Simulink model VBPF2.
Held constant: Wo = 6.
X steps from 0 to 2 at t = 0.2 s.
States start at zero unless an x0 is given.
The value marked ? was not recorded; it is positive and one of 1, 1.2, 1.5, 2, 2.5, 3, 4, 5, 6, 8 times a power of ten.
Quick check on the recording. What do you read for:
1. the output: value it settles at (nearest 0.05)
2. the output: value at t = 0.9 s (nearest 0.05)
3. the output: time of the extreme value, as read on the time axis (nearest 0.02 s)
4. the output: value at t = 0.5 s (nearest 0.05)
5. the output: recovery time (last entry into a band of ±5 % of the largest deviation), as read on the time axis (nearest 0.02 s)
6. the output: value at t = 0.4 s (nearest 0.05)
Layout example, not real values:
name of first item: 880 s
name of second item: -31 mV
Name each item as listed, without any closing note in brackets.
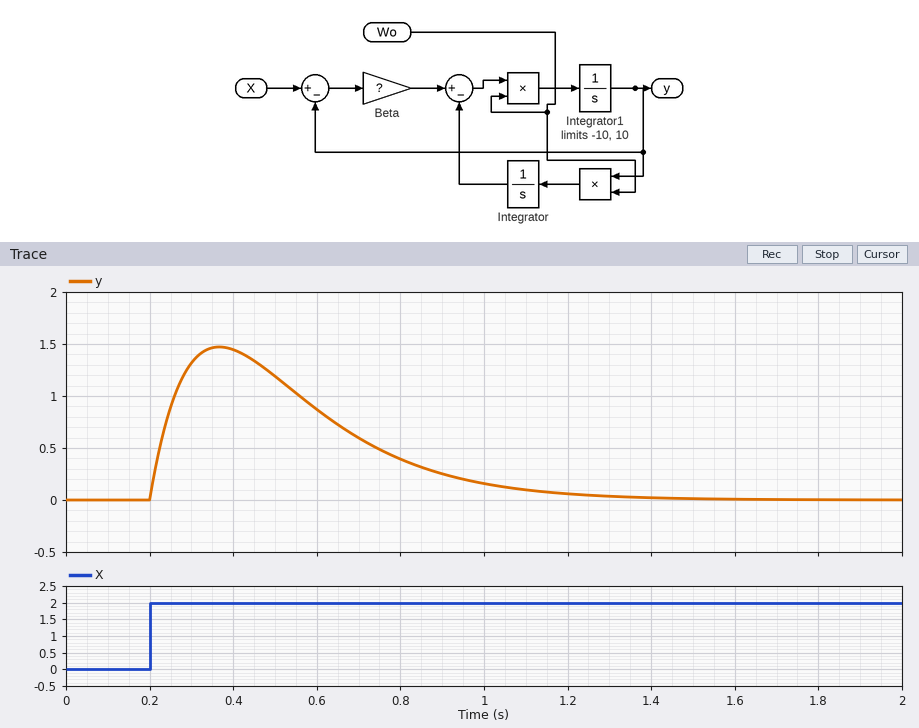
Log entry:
the output: value it settles at: 0.00
the output: value at t = 0.9 s: 0.25
the output: time of the extreme value, as read on the time axis: 0.36 s
the output: value at t = 0.5 s: 1.20
the output: recovery time (last entry into a band of ±5 % of the largest deviation), as read on the time axis: 1.16 s
the output: value at t = 0.4 s: 1.45
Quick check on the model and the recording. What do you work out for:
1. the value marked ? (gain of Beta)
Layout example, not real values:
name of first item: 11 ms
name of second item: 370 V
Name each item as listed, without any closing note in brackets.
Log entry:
the value marked ?: 2
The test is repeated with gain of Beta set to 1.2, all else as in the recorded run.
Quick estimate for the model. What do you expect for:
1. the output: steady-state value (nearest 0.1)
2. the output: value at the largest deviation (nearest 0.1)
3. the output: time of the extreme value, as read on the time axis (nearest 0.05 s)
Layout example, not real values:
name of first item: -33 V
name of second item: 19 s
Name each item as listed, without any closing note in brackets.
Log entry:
the output: steady-state value: 0.0
the output: value at the largest deviation: 1.2
the output: time of the extreme value, as read on the time axis: 0.40 s
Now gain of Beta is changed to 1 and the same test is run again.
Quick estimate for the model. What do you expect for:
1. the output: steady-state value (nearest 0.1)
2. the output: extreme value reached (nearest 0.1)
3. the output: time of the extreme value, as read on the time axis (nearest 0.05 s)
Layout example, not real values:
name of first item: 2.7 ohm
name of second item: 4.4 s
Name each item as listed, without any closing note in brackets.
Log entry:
the output: steady-state value: 0.0
the output: extreme value reached: 1.1
the output: time of the extreme value, as read on the time axis: 0.40 s
